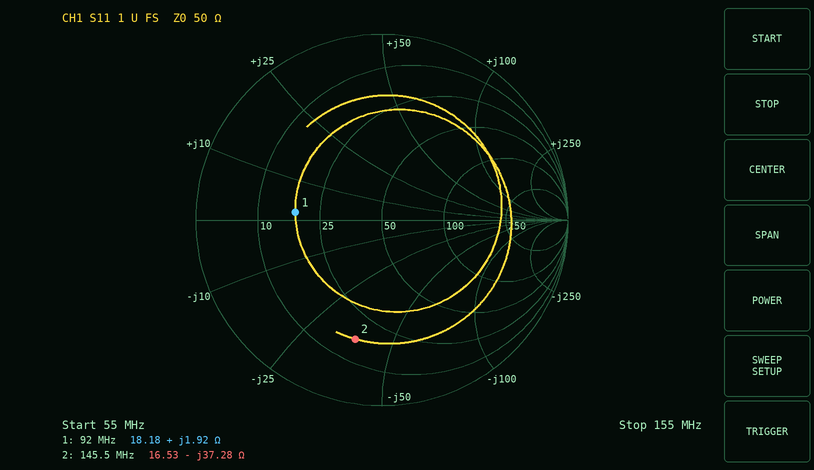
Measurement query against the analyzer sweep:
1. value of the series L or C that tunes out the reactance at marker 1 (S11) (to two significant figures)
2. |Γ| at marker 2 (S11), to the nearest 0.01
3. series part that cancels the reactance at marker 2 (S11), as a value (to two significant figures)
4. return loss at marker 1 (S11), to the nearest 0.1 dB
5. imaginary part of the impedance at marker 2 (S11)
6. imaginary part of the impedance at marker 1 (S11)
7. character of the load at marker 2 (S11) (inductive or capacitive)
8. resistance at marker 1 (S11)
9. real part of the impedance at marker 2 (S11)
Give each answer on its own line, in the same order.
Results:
900 pF
0.66
41 nH
6.6 dB
-37.28 Ω
+1.92 Ω
capacitive
18.18 Ω
16.53 Ω
